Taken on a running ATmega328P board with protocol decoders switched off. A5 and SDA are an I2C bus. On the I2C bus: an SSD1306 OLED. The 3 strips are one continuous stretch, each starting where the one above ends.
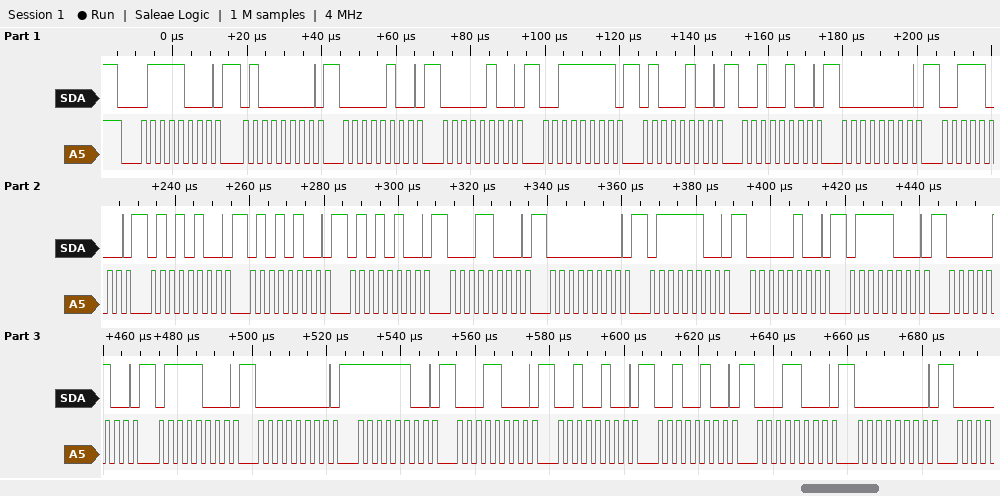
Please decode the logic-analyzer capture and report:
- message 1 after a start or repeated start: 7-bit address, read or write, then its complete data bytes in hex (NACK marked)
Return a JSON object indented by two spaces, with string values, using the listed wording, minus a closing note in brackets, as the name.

{
  "message 1 after a start or repeated start: 7-bit address, read or write, then its complete data bytes in hex": "0x3C write: 40 04 04 3F 44 24 00 38 54 54 54 18 00 7C 04 78 04 78 00 FC 18 24 24 18 00"
}
